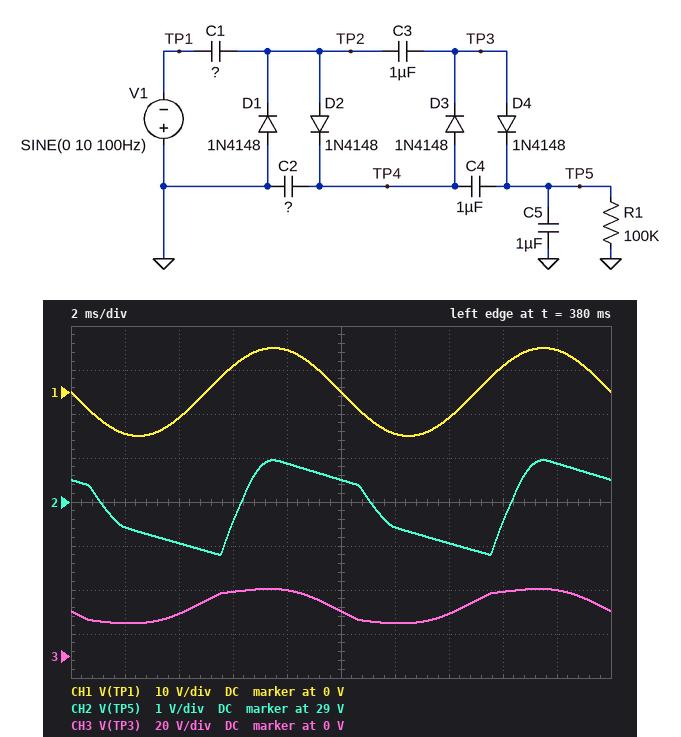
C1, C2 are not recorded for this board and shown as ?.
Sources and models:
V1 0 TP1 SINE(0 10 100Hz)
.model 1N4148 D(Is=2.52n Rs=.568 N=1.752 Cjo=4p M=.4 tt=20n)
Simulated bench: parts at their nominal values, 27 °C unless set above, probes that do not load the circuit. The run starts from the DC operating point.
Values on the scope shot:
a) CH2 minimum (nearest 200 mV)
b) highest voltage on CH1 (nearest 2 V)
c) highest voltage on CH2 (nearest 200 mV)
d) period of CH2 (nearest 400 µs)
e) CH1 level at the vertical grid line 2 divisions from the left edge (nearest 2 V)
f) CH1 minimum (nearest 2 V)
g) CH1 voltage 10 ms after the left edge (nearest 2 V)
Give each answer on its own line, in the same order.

27.8 V
10 V
30.0 V
10.0 ms
-6 V
-10 V
0 V
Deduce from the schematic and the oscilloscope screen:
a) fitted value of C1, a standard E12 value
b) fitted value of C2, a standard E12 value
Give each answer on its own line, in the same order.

3.3 µF
1.5 µF
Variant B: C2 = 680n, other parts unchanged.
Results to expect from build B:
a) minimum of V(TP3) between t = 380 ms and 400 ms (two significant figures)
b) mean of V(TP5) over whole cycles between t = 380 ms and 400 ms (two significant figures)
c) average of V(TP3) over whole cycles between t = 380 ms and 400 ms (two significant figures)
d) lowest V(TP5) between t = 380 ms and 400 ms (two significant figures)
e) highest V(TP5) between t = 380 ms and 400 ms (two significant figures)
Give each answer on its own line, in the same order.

14 V
28 V
22 V
26 V
29 V
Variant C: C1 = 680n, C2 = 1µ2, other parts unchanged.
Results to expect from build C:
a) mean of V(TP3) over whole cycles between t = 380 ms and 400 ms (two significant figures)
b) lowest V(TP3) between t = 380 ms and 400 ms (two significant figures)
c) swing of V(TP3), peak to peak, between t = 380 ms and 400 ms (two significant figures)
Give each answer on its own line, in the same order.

17 V
11 V
12 V
